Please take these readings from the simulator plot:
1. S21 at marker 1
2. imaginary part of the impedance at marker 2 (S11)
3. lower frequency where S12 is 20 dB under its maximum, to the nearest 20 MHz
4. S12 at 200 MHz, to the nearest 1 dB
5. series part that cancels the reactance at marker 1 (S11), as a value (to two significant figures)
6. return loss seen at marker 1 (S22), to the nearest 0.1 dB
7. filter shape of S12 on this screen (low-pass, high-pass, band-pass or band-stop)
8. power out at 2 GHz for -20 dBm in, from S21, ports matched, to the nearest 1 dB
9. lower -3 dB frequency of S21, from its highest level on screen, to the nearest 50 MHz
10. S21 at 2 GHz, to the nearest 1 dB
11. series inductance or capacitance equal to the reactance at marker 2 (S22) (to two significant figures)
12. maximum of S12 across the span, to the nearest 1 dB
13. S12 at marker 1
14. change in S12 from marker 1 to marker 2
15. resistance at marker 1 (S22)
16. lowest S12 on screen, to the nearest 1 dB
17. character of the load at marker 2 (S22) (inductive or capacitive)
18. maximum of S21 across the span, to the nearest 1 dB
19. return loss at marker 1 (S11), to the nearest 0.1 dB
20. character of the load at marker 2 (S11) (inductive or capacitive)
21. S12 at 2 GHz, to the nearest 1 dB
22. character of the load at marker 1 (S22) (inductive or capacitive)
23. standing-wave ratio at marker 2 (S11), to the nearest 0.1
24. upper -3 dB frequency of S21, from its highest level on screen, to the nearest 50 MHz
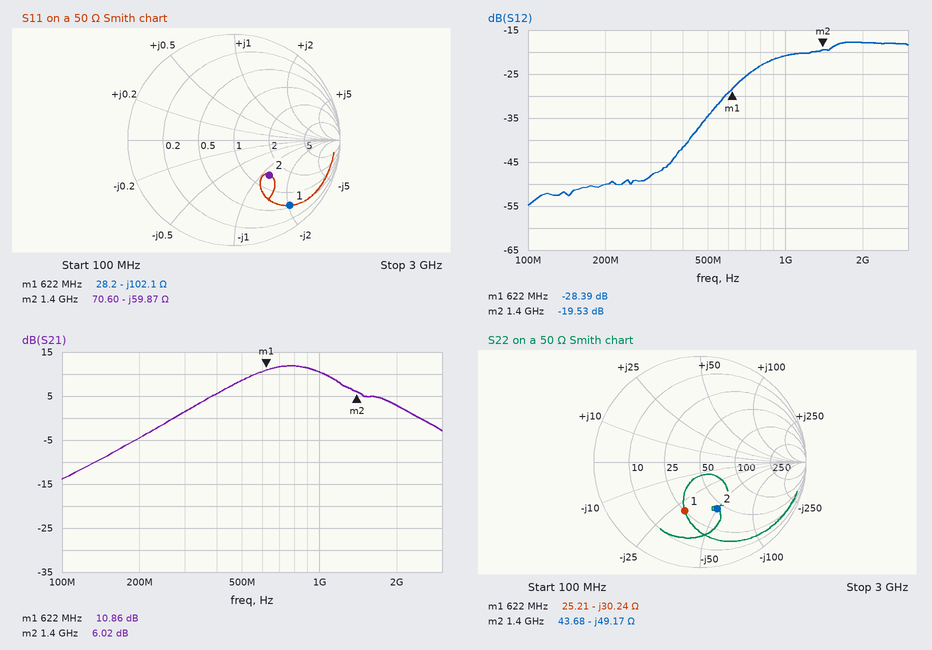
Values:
10.86 dB
-59.87 Ω
460 MHz
-50 dB
26 nH
6.3 dB
high-pass
-17 dBm
500 MHz
3 dB
2.3 pF
-18 dB
-28.39 dB
8.86 dB
25.21 Ω
-55 dB
capacitive
12 dB
1.8 dB
capacitive
-18 dB
capacitive
2.8
1.15 GHz
